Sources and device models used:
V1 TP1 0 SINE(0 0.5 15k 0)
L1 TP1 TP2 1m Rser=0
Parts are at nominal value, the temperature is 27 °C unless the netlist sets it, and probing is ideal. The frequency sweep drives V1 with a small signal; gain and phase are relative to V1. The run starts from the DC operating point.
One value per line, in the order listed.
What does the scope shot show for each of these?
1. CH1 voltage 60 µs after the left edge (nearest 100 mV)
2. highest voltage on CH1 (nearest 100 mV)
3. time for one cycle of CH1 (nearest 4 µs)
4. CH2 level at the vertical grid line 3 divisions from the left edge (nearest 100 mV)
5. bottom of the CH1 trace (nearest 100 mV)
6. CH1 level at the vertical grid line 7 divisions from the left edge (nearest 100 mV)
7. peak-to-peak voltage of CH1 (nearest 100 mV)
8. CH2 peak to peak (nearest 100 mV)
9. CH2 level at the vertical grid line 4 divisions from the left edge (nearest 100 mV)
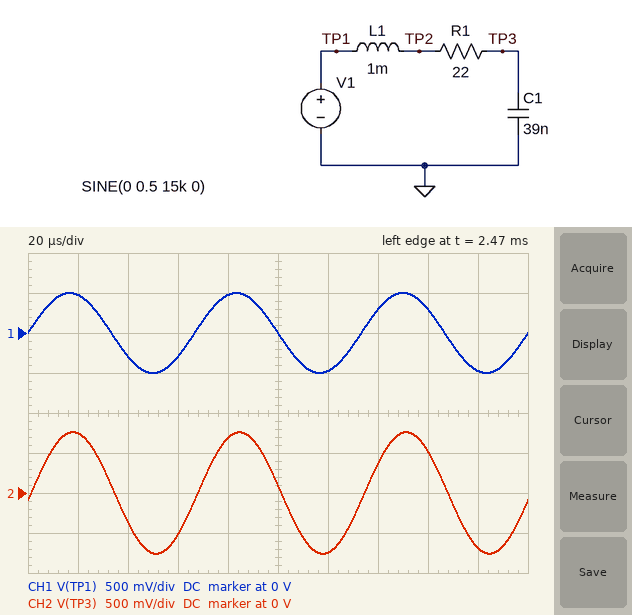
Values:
-300 mV
500 mV
68 µs
-500 mV
-500 mV
300 mV
1.0 V
1.5 V
700 mV
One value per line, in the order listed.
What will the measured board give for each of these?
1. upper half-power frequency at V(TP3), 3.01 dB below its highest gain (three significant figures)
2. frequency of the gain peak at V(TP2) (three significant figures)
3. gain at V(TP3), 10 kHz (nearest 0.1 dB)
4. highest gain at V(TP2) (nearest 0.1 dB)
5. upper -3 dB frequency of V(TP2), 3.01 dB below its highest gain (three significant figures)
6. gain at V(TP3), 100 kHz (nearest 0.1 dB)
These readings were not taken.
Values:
27.1 kHz
25.4 kHz
1.4 dB
17.3 dB
27.1 kHz
-23.2 dB
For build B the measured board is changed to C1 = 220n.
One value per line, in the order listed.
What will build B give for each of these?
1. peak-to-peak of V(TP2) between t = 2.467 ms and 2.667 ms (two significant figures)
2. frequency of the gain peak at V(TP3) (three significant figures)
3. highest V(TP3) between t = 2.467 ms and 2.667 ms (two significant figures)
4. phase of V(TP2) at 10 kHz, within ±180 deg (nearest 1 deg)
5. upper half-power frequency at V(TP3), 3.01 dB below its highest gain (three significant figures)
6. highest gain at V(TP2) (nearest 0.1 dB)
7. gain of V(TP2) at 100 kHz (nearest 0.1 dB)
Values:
1.0 V
10.4 kHz
470 mV
-50 deg
12.1 kHz
10.3 dB
-28.6 dB
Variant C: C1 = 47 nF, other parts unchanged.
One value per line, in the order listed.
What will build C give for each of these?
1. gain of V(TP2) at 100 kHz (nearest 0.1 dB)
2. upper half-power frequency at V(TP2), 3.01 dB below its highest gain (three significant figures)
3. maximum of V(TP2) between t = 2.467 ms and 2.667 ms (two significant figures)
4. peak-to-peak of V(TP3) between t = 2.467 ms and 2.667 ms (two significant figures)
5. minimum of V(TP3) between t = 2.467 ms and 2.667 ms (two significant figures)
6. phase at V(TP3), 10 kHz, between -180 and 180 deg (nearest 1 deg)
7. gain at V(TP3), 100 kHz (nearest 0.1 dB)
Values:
-23.4 dB
24.8 kHz
850 mV
1.7 V
-850 mV
-5 deg
-24.9 dB
